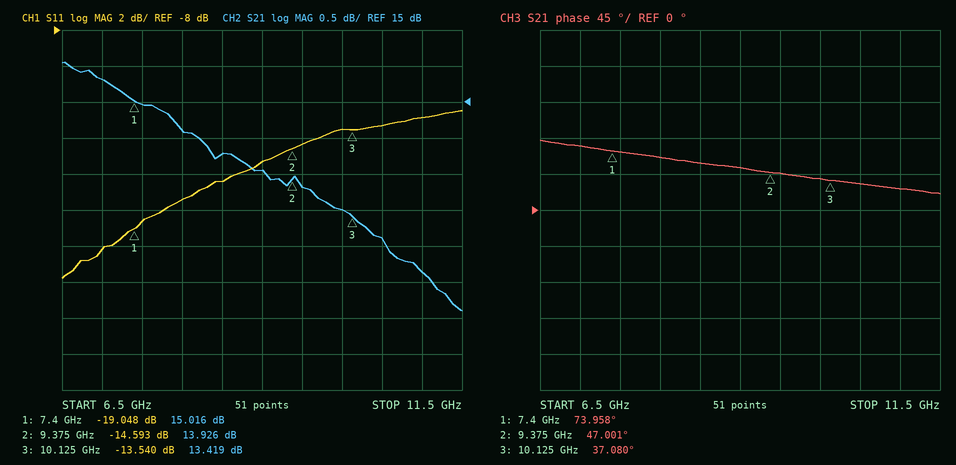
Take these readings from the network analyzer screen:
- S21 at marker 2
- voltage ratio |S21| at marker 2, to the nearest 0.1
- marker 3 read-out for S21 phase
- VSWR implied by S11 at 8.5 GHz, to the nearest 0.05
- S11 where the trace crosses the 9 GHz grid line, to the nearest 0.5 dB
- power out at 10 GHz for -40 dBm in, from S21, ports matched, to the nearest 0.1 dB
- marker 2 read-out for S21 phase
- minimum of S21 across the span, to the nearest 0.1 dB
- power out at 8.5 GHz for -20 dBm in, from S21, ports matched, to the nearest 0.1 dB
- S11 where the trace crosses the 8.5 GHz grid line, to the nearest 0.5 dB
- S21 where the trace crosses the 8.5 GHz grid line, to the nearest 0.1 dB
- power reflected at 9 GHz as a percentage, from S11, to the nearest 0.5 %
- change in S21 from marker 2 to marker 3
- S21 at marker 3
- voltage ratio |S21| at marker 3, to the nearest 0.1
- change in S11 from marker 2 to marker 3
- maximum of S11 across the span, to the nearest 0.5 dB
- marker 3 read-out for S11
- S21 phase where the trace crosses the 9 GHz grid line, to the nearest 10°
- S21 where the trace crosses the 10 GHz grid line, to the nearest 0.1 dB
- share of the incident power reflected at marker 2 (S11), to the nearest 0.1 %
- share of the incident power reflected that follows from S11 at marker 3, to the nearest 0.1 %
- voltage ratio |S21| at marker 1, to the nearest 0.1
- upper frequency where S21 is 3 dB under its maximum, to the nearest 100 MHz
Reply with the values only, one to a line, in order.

13.926 dB
5.0
37.080°
1.35
-15.5 dB
-26.5 dBm
47.001°
12.1 dB
-5.7 dBm
-16.5 dB
14.3 dB
3.0 %
-0.507 dB
13.419 dB
4.7
1.053 dB
-12.5 dB
-13.540 dB
50°
13.5 dB
3.5 %
4.4 %
5.6
11.1 GHz
